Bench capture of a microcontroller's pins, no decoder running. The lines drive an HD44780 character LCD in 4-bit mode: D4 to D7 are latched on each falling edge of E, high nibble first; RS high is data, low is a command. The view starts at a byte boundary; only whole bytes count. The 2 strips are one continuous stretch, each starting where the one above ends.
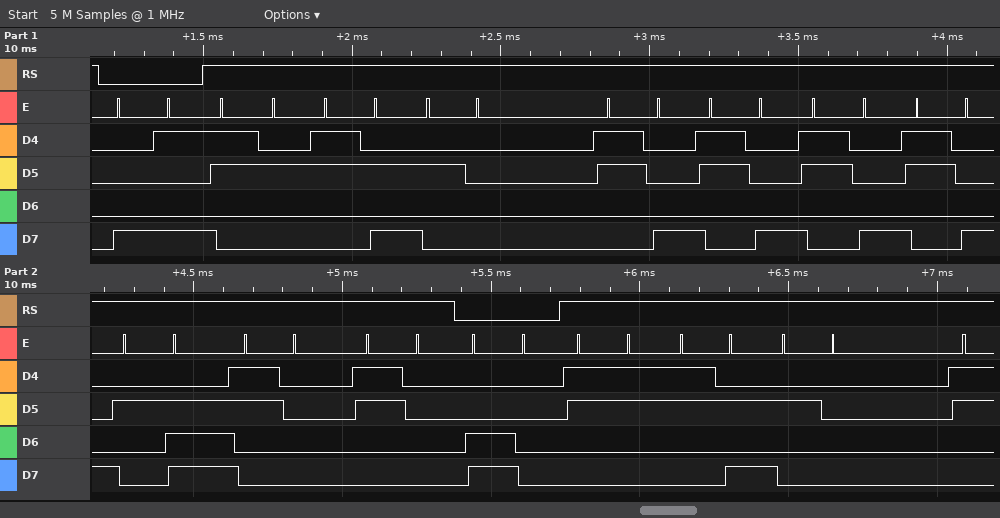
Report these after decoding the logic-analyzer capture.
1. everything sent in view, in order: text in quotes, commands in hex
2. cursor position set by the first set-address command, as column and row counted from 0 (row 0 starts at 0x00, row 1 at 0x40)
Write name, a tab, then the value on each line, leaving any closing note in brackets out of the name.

everything sent in view, in order: text in quotes, commands in hex	0x89 "2: 8888.00" 0xC0 "3: "
cursor position set by the first set-address command, as column and row counted from 0	column 9, row 0
